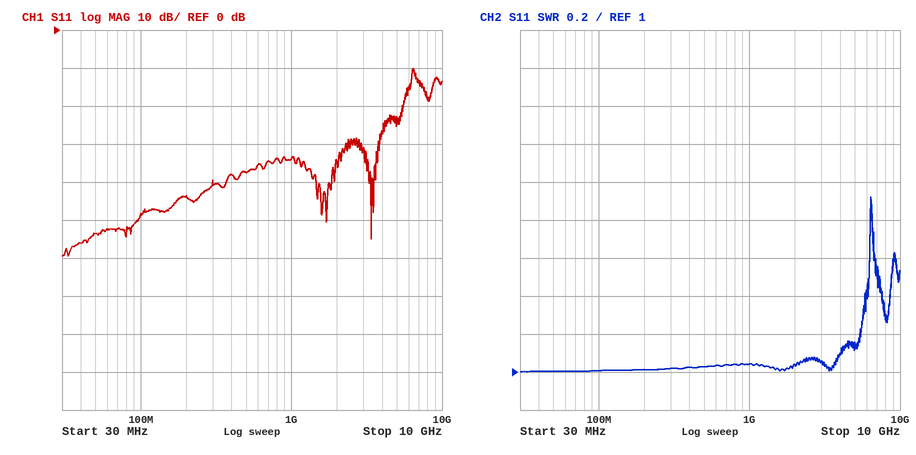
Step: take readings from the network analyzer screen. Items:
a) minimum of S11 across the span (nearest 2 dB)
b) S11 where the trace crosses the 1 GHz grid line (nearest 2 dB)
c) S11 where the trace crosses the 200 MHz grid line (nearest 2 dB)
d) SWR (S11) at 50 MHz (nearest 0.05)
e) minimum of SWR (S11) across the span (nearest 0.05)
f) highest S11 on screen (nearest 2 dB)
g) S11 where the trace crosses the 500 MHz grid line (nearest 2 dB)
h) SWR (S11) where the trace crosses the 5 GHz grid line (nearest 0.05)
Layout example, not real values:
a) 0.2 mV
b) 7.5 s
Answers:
a) -60 dB
b) -34 dB
c) -44 dB
d) 1.00
e) 1.00
f) -10 dB
g) -38 dB
h) 1.15
